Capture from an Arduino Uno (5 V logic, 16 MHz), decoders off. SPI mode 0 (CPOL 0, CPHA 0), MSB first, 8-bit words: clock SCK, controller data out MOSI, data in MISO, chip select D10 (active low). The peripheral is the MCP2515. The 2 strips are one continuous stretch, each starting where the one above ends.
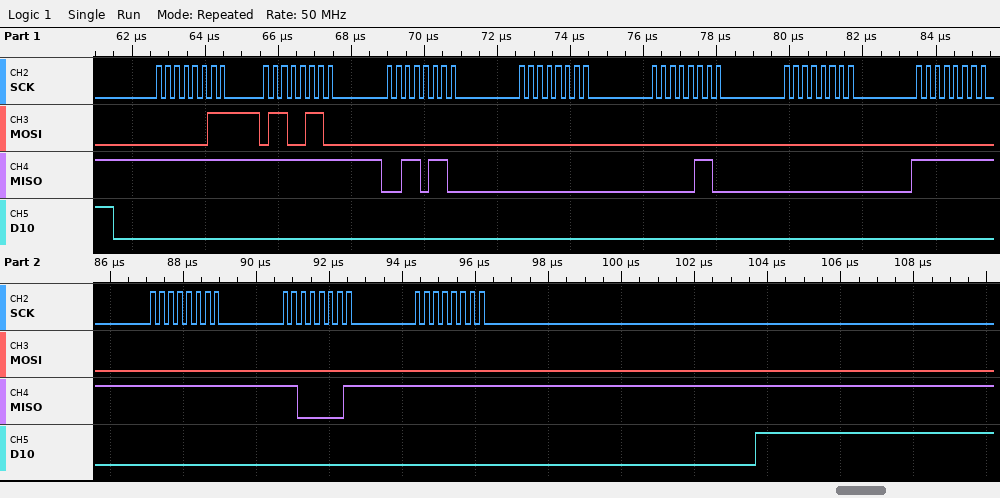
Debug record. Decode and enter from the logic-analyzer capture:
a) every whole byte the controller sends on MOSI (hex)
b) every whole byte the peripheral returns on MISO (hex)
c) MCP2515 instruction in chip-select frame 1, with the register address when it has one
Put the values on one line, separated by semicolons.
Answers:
03 66 00 00 00 00 00 00 00 00; FF FF 36 00 06 00 FF FF C1 FF; READ 0x66
